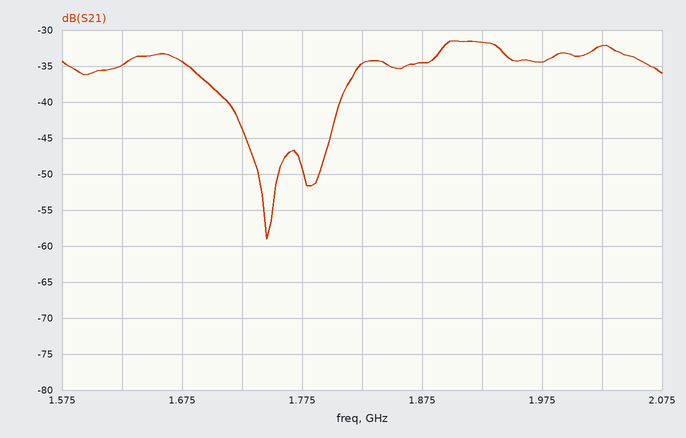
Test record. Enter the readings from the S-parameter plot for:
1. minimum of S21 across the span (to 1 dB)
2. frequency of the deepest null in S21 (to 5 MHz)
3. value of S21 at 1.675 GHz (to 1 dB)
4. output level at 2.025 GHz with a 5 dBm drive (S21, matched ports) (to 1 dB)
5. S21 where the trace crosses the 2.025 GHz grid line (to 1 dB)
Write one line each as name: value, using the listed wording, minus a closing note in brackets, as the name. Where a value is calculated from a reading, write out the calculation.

minimum of S21 across the span: -59 dB
frequency of the deepest null in S21: 1.745 GHz
value of S21 at 1.675 GHz: -34 dB
output level at 2.025 GHz with a 5 dBm drive (S21, matched ports): 5 dBm + (-32 dB) = -27 dBm
S21 where the trace crosses the 2.025 GHz grid line: -32 dB
